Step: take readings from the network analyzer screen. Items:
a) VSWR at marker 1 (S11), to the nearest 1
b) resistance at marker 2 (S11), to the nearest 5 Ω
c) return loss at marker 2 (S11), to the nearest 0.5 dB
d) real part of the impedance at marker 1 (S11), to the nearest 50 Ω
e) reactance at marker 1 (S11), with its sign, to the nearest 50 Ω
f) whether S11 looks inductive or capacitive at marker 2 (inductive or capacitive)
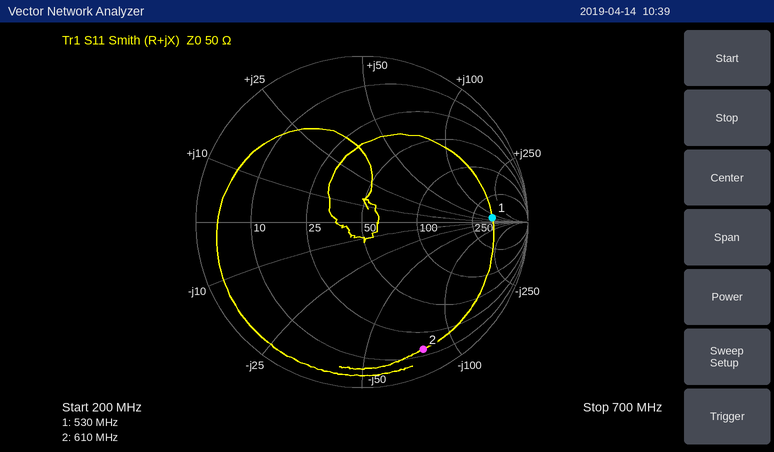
8
15 Ω
1.5 dB
400 Ω
+50 Ω
capacitive
